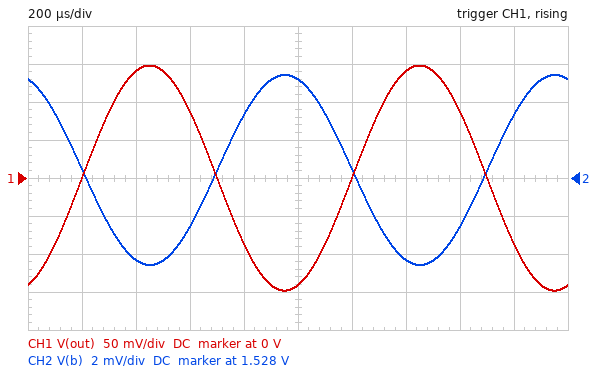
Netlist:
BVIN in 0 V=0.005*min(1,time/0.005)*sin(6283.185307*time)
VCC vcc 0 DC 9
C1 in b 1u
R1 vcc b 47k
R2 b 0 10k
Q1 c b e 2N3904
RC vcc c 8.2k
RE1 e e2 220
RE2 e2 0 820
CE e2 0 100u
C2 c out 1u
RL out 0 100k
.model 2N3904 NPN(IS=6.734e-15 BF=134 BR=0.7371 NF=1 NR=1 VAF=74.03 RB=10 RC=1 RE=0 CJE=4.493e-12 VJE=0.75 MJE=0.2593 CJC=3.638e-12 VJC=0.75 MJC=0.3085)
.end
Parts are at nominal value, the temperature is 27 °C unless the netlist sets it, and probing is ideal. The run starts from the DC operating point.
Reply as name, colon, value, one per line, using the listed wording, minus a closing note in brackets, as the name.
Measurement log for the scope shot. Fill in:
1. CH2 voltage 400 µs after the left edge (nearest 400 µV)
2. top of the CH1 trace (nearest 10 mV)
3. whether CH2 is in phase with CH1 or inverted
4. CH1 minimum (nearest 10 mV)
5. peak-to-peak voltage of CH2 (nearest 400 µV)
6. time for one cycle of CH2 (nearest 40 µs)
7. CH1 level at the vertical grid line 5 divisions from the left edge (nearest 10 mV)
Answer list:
CH2 voltage 400 µs after the left edge: 1.5236 V
top of the CH1 trace: 150 mV
whether CH2 is in phase with CH1 or inverted: inverted
CH1 minimum: -150 mV
peak-to-peak voltage of CH2: 10.0 mV
time for one cycle of CH2: 1.00 ms
CH1 level at the vertical grid line 5 divisions from the left edge: -140 mV
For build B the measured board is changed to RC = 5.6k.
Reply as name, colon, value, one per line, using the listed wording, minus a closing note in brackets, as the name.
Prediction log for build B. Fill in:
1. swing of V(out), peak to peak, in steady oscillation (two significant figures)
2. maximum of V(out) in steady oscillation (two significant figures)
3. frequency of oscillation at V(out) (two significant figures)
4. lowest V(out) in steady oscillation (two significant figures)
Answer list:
swing of V(out), peak to peak, in steady oscillation: 210 mV
maximum of V(out) in steady oscillation: 100 mV
frequency of oscillation at V(out): 1.0 kHz
lowest V(out) in steady oscillation: -100 mV
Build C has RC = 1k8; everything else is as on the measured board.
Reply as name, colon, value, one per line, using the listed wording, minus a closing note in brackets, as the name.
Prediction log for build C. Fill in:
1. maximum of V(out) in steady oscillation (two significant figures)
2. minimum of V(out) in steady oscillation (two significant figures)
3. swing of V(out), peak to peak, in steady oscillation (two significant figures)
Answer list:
maximum of V(out) in steady oscillation: 35 mV
minimum of V(out) in steady oscillation: -35 mV
swing of V(out), peak to peak, in steady oscillation: 70 mV
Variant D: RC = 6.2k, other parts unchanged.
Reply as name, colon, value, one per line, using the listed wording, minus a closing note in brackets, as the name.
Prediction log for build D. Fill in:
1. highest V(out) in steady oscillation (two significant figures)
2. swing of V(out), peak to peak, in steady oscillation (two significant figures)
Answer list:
highest V(out) in steady oscillation: 110 mV
swing of V(out), peak to peak, in steady oscillation: 230 mV
